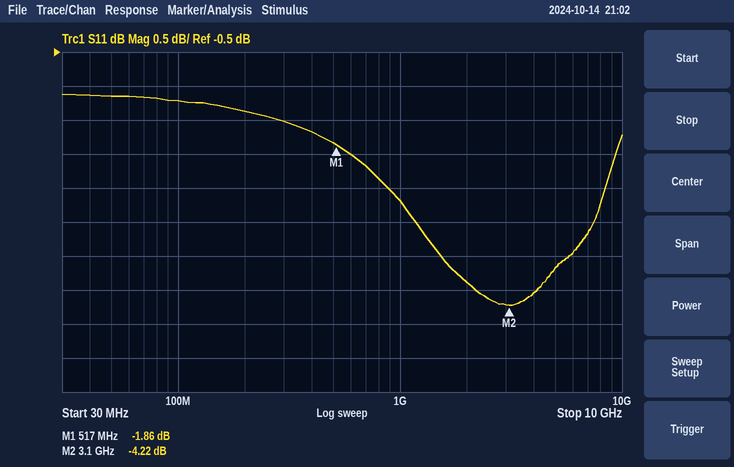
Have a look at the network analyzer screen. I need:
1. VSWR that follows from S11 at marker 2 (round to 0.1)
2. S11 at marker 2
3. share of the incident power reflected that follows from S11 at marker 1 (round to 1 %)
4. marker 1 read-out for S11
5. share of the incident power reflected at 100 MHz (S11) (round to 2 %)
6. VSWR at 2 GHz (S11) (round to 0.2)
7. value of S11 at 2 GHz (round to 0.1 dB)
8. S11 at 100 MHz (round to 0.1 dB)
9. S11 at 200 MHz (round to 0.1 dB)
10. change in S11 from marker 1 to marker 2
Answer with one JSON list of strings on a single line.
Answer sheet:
["4.2", "-4.22 dB", "65 %", "-1.86 dB", "76 %", "4.6", "-3.9 dB", "-1.2 dB", "-1.4 dB", "-2.36 dB"]
